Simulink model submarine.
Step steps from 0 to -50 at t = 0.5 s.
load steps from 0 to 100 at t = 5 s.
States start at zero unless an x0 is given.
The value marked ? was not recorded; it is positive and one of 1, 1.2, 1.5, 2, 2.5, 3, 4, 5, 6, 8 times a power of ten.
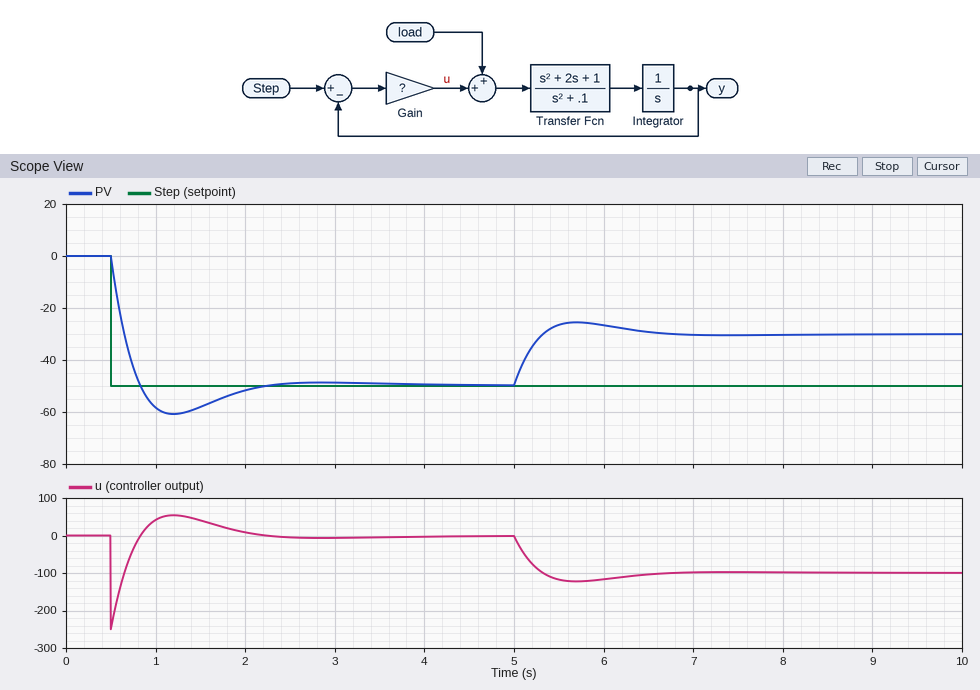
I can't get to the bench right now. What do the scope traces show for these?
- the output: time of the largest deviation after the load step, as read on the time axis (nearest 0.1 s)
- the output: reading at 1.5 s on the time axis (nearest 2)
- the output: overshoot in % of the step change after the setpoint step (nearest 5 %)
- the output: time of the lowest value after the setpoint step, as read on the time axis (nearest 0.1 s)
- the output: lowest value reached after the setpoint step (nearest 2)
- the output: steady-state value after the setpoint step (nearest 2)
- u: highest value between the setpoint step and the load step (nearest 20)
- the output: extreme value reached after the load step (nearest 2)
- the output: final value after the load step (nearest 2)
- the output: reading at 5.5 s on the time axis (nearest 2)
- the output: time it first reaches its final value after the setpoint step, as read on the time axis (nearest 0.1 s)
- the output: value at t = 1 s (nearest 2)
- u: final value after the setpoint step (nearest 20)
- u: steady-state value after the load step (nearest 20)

5.7 s
-58
20 %
1.2 s
-60
-50
60
-26
-30
-26
0.8 s
-58
0
-100
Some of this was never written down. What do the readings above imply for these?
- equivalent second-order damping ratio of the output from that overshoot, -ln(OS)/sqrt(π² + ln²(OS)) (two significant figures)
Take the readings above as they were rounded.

0.46
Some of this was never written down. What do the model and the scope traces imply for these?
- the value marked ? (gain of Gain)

5
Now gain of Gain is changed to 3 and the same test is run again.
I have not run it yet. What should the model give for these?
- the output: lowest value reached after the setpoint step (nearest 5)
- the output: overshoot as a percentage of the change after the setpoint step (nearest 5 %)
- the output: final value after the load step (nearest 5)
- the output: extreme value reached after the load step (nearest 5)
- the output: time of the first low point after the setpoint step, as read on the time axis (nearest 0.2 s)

-65
30 %
-15
-5
1.4 s
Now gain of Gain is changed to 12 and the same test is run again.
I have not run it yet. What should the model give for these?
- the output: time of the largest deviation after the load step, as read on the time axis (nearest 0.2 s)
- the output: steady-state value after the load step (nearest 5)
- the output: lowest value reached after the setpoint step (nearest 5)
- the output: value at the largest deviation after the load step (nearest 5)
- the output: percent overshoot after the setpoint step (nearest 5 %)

5.4 s
-40
-55
-40
10 %
